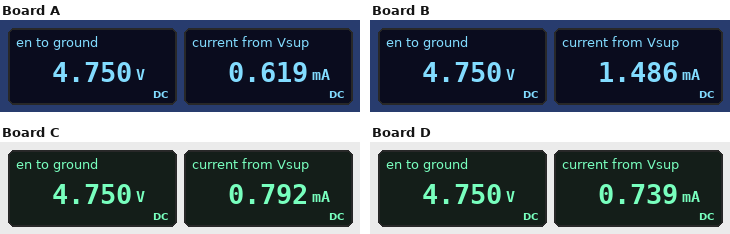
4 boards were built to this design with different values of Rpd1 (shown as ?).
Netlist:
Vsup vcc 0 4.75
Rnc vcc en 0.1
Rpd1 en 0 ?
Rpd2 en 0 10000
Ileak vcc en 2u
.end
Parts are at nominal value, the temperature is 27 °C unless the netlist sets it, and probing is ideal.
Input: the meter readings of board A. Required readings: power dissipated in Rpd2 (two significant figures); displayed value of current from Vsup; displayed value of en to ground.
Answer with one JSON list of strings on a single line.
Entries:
["2.3 mW", "0.619 mA", "4.750 V"]
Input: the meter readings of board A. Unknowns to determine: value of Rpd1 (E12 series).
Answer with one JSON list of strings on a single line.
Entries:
["33 kΩ"]
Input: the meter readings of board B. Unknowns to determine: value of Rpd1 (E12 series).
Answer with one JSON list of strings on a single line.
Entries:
["4.7 kΩ"]
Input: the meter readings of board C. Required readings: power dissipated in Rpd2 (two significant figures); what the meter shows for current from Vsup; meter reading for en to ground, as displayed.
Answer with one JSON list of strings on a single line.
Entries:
["2.3 mW", "0.792 mA", "4.750 V"]
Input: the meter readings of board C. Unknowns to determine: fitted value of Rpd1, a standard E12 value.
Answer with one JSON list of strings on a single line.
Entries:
["15 kΩ"]
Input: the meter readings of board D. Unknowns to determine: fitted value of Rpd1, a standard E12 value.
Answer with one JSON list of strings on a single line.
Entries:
["18 kΩ"]
